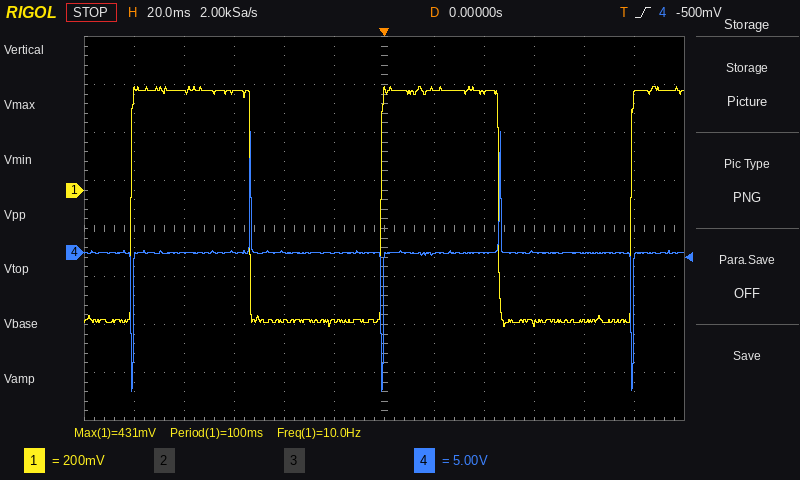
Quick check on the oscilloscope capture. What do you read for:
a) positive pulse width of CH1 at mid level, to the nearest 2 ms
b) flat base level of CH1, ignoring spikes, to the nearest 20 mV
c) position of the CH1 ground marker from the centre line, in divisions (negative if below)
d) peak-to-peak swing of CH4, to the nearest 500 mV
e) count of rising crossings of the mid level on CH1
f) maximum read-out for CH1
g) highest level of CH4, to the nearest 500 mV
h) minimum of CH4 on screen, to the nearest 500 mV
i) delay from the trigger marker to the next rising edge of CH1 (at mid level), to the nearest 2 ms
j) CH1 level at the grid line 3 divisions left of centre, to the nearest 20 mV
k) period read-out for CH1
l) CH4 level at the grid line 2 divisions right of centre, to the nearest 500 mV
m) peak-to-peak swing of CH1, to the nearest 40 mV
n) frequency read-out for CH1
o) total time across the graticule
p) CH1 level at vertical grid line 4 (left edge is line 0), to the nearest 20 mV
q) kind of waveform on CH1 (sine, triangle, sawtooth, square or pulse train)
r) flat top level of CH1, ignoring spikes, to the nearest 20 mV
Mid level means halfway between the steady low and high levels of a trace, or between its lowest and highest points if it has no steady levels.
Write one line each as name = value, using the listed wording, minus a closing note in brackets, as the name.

positive pulse width of CH1 at mid level, to the nearest 2 ms = 48 ms
flat base level of CH1, ignoring spikes, to the nearest 20 mV = -540 mV
position of the CH1 ground marker from the centre line, in divisions = +0.8 div
peak-to-peak swing of CH4, to the nearest 500 mV = 27.0 V
count of rising crossings of the mid level on CH1 = 3
maximum read-out for CH1 = 431 mV
highest level of CH4, to the nearest 500 mV = 12.5 V
minimum of CH4 on screen, to the nearest 500 mV = -14.5 V
delay from the trigger marker to the next rising edge of CH1 (at mid level), to the nearest 2 ms = 98 ms
CH1 level at the grid line 3 divisions left of centre, to the nearest 20 mV = 400 mV
period read-out for CH1 = 100 ms
CH4 level at the grid line 2 divisions right of centre, to the nearest 500 mV = 0.0 V
peak-to-peak swing of CH1, to the nearest 40 mV = 1.00 V
frequency read-out for CH1 = 10.0 Hz
total time across the graticule = 240 ms
CH1 level at vertical grid line 4 (left edge is line 0), to the nearest 20 mV = -540 mV
kind of waveform on CH1 = square
flat top level of CH1, ignoring spikes, to the nearest 20 mV = 420 mV
